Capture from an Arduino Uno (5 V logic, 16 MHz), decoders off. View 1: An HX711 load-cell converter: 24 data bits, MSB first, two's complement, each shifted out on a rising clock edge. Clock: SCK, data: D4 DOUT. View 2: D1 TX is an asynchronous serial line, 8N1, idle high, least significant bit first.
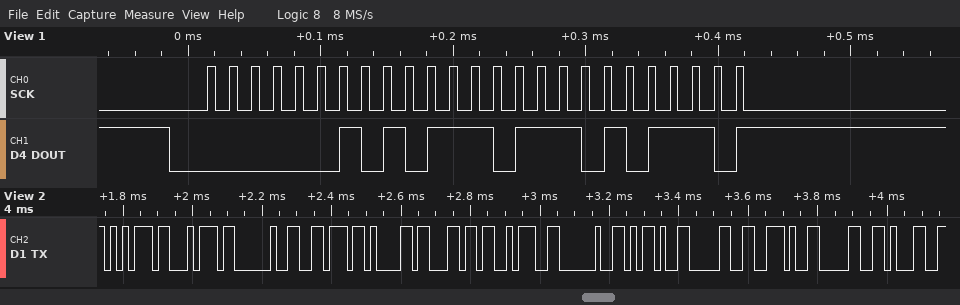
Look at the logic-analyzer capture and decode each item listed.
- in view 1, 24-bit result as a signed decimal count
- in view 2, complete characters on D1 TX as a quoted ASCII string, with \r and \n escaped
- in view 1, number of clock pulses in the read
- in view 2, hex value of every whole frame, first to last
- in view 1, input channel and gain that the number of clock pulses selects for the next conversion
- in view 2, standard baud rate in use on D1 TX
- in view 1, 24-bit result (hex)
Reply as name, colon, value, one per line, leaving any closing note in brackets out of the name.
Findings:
in view 1, 24-bit result as a signed decimal count: 179118
in view 2, complete characters on D1 TX as a quoted ASCII string, with \r and \n escaped: "ut val: -0.01"
in view 1, number of clock pulses in the read: 25
in view 2, hex value of every whole frame, first to last: 0x75 0x74 0x20 0x76 0x61 0x6C 0x3A 0x20 0x2D 0x30 0x2E 0x30 0x31
in view 1, input channel and gain that the number of clock pulses selects for the next conversion: channel A, gain 128
in view 2, standard baud rate in use on D1 TX: 57600 baud
in view 1, 24-bit result: 0x02BBAE
